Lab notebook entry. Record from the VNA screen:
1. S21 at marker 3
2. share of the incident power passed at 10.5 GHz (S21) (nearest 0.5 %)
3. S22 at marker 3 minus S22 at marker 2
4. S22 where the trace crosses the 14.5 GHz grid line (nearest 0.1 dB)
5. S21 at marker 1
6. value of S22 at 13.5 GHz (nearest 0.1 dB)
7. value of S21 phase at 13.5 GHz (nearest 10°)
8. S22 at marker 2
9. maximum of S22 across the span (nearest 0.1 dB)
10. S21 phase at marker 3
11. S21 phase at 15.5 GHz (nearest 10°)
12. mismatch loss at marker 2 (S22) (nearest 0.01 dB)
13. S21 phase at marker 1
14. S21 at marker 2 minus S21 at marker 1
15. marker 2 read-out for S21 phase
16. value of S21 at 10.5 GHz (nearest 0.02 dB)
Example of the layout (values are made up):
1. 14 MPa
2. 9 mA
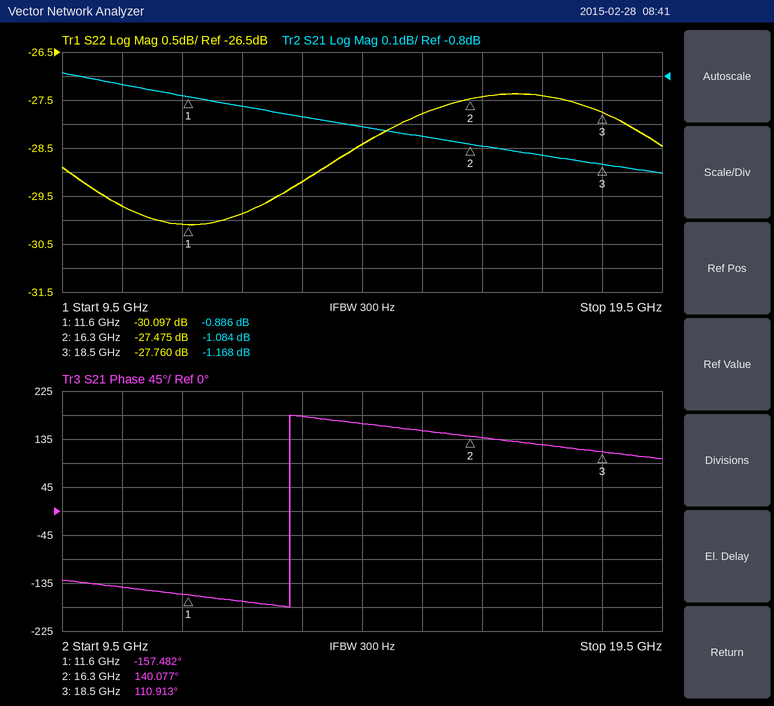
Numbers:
1. -1.168 dB
2. 82.5 %
3. -0.285 dB
4. -28.4 dB
5. -0.886 dB
6. -29.2 dB
7. 180°
8. -27.475 dB
9. -27.4 dB
10. 110.913°
11. 150°
12. 0.01 dB
13. -157.482°
14. -0.198 dB
15. 140.077°
16. -0.84 dB
